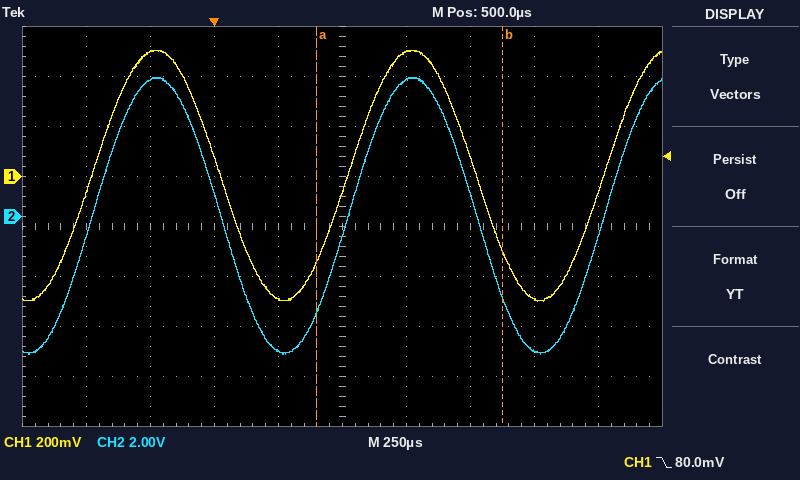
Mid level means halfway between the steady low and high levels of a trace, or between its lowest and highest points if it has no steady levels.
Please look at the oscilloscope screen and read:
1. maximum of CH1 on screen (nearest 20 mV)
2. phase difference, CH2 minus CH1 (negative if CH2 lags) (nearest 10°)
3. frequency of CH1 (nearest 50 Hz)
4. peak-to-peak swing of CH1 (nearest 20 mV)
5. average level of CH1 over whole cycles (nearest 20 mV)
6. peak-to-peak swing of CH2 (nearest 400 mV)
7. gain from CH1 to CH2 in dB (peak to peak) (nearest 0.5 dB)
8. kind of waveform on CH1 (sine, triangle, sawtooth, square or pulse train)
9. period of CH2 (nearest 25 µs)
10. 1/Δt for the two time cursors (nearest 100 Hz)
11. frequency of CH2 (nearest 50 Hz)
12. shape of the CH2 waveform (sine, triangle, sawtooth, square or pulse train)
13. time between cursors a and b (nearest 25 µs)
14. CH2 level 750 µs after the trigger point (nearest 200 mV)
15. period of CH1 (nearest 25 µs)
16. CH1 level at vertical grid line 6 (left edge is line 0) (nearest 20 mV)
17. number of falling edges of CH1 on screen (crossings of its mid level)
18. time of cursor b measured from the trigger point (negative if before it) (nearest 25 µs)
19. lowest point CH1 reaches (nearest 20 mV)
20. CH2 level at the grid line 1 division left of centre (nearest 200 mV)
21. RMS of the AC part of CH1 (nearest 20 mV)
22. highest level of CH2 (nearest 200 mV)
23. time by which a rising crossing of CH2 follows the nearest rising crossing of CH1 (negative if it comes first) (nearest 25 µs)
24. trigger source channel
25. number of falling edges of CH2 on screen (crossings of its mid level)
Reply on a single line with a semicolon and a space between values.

500 mV; 0°; 1.00 kHz; 1.00 V; 0 mV; 11.2 V; 21.0 dB; sine; 1.000 ms; 1.4 kHz; 1.00 kHz; sine; 725 µs; 5.4 V; 1.000 ms; 500 mV; 2; +1.125 ms; -500 mV; -5.4 V; 360 mV; 5.6 V; 0 µs; CH1; 2
